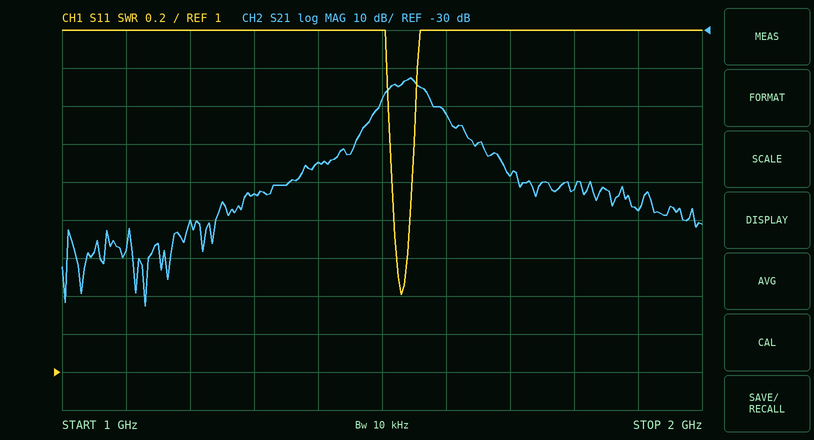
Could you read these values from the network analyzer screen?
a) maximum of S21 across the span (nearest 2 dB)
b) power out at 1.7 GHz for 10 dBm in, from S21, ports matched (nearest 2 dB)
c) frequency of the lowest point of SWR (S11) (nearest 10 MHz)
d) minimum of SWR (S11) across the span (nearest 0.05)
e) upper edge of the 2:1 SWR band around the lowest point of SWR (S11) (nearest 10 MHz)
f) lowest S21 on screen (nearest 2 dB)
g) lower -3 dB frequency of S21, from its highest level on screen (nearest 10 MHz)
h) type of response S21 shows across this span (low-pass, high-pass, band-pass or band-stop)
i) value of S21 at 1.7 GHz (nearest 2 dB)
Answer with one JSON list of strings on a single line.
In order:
["-42 dB", "-58 dBm", "1.53 GHz", "1.40", "1.55 GHz", "-102 dB", "1.51 GHz", "band-pass", "-68 dB"]
